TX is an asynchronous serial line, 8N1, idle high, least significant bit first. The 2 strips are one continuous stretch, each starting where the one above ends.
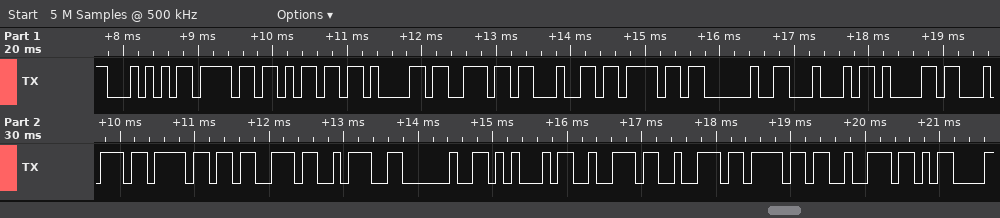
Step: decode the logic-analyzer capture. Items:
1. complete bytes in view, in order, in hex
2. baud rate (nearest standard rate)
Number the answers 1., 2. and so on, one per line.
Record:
1. 54 6F 6D 61 6E 64 6F 20 44 61 74 6F 73 3A 20 45 72 72 6F 72 0D
2. 9600 baud
